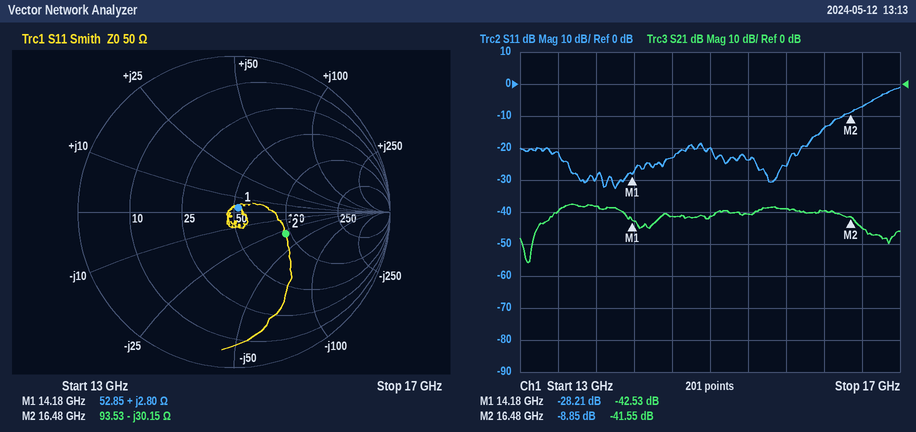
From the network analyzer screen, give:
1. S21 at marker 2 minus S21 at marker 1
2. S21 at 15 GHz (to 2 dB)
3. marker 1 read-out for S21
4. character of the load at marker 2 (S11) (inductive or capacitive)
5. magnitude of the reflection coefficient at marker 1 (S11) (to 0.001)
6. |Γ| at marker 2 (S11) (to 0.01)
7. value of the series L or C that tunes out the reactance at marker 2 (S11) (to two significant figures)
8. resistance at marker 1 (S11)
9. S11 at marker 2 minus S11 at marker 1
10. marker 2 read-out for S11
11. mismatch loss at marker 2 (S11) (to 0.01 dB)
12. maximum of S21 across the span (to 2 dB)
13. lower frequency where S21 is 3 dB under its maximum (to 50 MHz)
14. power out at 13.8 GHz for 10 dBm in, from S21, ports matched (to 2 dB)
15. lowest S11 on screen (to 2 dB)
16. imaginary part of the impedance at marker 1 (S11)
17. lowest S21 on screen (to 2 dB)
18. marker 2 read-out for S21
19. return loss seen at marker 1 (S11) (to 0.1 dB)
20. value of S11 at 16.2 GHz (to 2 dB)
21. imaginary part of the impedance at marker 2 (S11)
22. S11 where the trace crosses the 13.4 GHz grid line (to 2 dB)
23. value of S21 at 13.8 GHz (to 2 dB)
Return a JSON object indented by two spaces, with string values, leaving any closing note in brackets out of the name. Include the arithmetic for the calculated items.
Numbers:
{
  "S21 at marker 2 minus S21 at marker 1": "-41.55 − (-42.53) = 0.98 dB",
  "S21 at 15 GHz": "-42 dB",
  "marker 1 read-out for S21": "-42.53 dB",
  "character of the load at marker 2 (S11)": "capacitive",
  "magnitude of the reflection coefficient at marker 1 (S11)": "10^(-28.21/20) ≈ 0.039",
  "|Γ| at marker 2 (S11)": "0.36",
  "value of the series L or C that tunes out the reactance at marker 2 (S11)": "L = 30.15 Ω/(2π × 16.48 GHz) ≈ 291 pH, so 290 pH to two significant figures",
  "resistance at marker 1": "52.85 Ω",
  "S11 at marker 2 minus S11 at marker 1": "-8.85 − (-28.21) = 19.36 dB",
  "marker 2 read-out for S11": "-8.85 dB",
  "mismatch loss at marker 2 (S11)": "−10 log10(1 − 10^(-8.85/10)) ≈ 0.61 dB",
  "maximum of S21 across the span": "-38 dB",
  "lower frequency where S21 is 3 dB under its maximum": "13.35 GHz",
  "power out at 13.8 GHz for 10 dBm in, from S21, ports matched": "10 dBm + (-38 dB) = -28 dBm",
  "lowest S11 on screen": "-32 dB",
  "imaginary part of the impedance at marker 1": "+2.80 Ω",
  "lowest S21 on screen": "-56 dB",
  "marker 2 read-out for S21": "-41.55 dB",
  "return loss seen at marker 1 (S11)": "28.2 dB",
  "value of S11 at 16.2 GHz": "-14 dB",
  "imaginary part of the impedance at marker 2": "-30.15 Ω",
  "S11 where the trace crosses the 13.4 GHz grid line": "-22 dB",
  "value of S21 at 13.8 GHz": "-38 dB"
}
